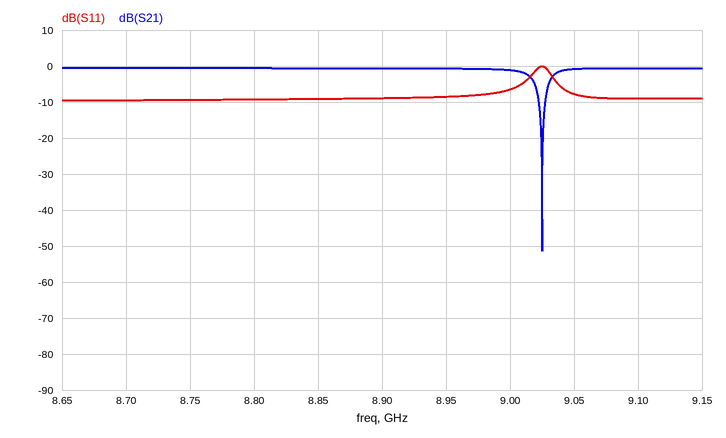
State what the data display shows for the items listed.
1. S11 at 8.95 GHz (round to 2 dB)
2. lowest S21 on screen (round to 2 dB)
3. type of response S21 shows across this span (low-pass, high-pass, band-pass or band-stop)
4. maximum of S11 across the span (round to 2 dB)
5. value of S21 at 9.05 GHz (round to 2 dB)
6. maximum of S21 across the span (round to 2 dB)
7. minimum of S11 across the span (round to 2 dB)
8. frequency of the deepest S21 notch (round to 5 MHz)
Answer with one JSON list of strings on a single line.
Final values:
["-8 dB", "-52 dB", "band-stop", "0 dB", "0 dB", "0 dB", "-10 dB", "9.025 GHz"]
